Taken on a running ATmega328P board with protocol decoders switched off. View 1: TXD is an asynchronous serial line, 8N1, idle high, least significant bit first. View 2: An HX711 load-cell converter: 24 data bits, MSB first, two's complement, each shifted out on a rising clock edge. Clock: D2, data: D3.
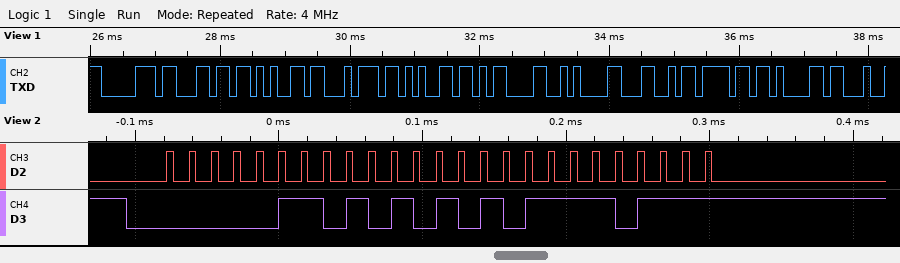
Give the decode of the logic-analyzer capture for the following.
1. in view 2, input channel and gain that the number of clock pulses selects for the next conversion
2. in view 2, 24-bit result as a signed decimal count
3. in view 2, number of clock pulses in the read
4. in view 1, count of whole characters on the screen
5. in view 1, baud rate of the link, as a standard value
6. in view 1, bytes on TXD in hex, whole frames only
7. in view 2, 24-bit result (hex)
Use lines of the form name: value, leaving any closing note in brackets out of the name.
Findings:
in view 2, input channel and gain that the number of clock pulses selects for the next conversion: channel A, gain 128
in view 2, 24-bit result as a signed decimal count: 436983
in view 2, number of clock pulses in the read: 25
in view 1, count of whole characters on the screen: 10
in view 1, baud rate of the link, as a standard value: 9600 baud
in view 1, bytes on TXD in hex, whole frames only: 0x70 0x6C 0x65 0x74 0x65 0x0D 0x0A 0x4C 0x6F 0x61
in view 2, 24-bit result: 0x06AAF7
